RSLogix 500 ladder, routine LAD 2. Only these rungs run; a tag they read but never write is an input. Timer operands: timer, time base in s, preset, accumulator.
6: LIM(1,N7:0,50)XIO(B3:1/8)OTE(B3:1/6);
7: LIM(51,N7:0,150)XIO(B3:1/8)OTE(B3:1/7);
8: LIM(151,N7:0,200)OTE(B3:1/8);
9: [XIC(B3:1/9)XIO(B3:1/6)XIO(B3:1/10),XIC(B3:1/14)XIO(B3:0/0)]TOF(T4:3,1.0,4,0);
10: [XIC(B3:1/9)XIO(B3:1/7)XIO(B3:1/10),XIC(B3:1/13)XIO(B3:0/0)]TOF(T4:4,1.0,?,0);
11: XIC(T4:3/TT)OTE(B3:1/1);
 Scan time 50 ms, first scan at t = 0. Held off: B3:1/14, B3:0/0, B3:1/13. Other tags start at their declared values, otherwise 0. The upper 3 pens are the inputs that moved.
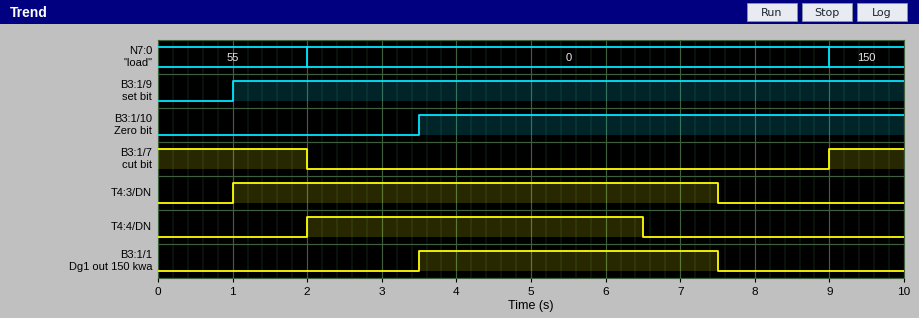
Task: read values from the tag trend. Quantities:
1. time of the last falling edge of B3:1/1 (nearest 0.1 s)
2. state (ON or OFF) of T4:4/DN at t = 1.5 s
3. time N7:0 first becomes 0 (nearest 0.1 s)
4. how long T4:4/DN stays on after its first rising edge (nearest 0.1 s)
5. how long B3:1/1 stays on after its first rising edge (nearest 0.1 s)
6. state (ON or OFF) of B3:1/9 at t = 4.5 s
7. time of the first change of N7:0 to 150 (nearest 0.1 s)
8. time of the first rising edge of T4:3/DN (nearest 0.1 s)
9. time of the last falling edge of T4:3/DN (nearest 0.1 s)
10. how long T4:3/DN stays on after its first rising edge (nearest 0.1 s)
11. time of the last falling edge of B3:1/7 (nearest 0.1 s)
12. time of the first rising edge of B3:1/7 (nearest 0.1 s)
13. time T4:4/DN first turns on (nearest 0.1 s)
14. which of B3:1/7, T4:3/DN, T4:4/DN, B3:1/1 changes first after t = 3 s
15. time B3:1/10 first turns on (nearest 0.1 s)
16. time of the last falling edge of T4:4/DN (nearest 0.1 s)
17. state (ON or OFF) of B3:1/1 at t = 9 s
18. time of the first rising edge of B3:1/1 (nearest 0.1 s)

7.5 s
OFF
2.0 s
4.5 s
4.0 s
ON
9.0 s
1.0 s
7.5 s
6.5 s
2.0 s
9.0 s
2.0 s
B3:1/1
3.5 s
6.5 s
OFF
3.5 s
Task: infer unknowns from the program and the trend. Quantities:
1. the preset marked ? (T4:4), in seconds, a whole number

3 s
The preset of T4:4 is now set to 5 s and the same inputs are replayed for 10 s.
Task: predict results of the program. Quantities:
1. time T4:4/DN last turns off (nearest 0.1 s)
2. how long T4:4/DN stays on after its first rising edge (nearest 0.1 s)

8.5 s
6.5 s
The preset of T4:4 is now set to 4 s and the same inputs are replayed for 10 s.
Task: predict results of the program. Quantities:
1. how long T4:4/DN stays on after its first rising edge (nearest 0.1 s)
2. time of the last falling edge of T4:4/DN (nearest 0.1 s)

5.5 s
7.5 s
